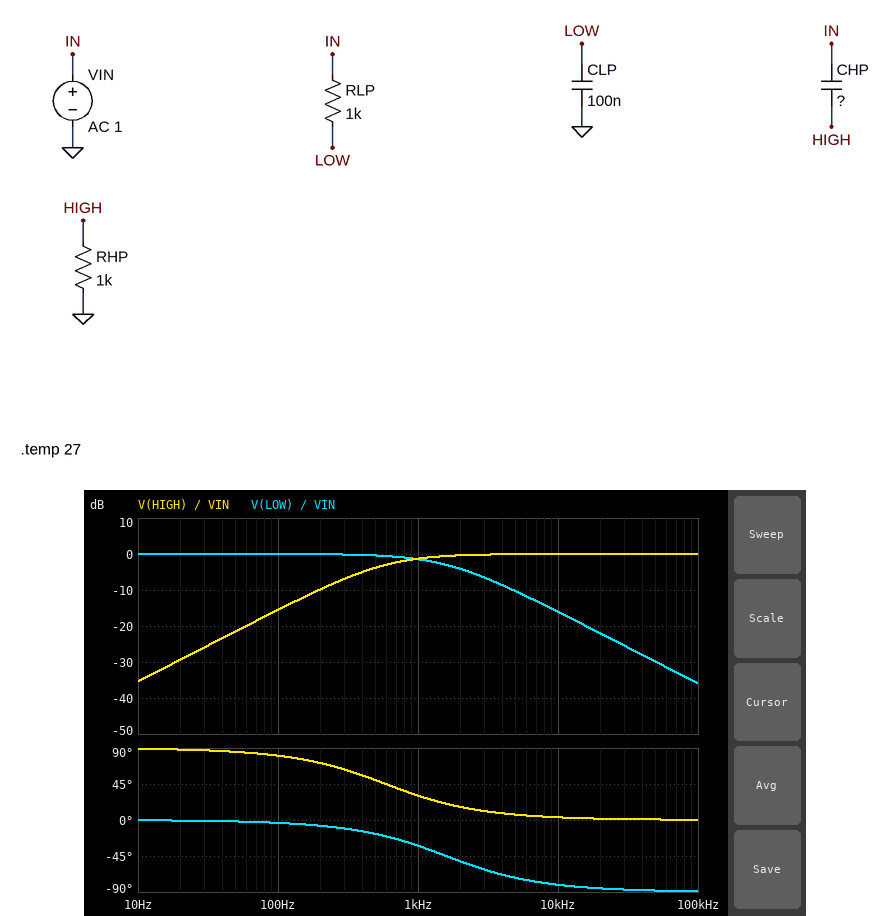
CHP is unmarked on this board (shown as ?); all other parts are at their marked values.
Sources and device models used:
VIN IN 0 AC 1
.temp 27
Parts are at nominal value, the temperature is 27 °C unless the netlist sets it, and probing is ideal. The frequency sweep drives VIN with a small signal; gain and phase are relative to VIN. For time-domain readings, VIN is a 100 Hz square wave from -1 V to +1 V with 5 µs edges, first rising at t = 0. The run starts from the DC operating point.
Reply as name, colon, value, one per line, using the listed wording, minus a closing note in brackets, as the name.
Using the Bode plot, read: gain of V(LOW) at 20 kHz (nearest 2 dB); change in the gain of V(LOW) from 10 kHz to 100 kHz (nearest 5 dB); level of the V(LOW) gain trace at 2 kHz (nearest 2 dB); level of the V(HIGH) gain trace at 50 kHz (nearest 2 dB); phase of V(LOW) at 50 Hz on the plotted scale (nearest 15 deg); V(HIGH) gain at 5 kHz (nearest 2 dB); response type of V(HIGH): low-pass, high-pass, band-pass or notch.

gain of V(LOW) at 20 kHz: -22 dB
change in the gain of V(LOW) from 10 kHz to 100 kHz: -20 dB
level of the V(LOW) gain trace at 2 kHz: -4 dB
level of the V(HIGH) gain trace at 50 kHz: 0 dB
phase of V(LOW) at 50 Hz on the plotted scale: 0 deg
V(HIGH) gain at 5 kHz: 0 dB
response type of V(HIGH): low-pass, high-pass, band-pass or notch: high-pass
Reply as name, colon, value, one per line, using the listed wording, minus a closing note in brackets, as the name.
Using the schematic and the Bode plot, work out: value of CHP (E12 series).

value of CHP: 270 nF
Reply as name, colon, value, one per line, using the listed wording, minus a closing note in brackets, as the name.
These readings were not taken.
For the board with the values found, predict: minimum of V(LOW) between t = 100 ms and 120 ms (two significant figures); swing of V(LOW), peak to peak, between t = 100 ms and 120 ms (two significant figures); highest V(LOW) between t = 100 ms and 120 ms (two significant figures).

minimum of V(LOW) between t = 100 ms and 120 ms: -1.0 V
swing of V(LOW), peak to peak, between t = 100 ms and 120 ms: 2.0 V
highest V(LOW) between t = 100 ms and 120 ms: 1.0 V
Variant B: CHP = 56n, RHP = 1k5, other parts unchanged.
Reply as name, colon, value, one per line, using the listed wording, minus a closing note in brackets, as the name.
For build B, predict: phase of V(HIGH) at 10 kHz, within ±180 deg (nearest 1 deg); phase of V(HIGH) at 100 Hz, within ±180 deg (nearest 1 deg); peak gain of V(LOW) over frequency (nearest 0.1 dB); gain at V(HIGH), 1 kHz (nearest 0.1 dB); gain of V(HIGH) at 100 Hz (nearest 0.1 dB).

phase of V(HIGH) at 10 kHz, within ±180 deg: 11 deg
phase of V(HIGH) at 100 Hz, within ±180 deg: 87 deg
peak gain of V(LOW) over frequency: 0 dB
gain at V(HIGH), 1 kHz: -6.6 dB
gain of V(HIGH) at 100 Hz: -25.6 dB
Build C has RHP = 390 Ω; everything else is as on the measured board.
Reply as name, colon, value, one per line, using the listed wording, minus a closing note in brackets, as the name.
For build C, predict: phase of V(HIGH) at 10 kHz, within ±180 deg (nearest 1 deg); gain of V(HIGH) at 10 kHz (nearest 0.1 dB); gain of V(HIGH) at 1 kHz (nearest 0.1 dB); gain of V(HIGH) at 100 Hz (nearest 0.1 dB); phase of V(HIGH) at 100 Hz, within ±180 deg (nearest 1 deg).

phase of V(HIGH) at 10 kHz, within ±180 deg: 9 deg
gain of V(HIGH) at 10 kHz: -0.1 dB
gain of V(HIGH) at 1 kHz: -5.2 dB
gain of V(HIGH) at 100 Hz: -23.6 dB
phase of V(HIGH) at 100 Hz, within ±180 deg: 86 deg
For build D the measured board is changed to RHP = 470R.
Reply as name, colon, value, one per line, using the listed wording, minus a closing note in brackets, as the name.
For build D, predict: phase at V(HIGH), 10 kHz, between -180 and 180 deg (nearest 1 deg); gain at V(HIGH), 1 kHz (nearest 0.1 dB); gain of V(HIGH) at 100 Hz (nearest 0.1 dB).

phase at V(HIGH), 10 kHz, between -180 and 180 deg: 7 deg
gain at V(HIGH), 1 kHz: -4.1 dB
gain of V(HIGH) at 100 Hz: -22.0 dB
